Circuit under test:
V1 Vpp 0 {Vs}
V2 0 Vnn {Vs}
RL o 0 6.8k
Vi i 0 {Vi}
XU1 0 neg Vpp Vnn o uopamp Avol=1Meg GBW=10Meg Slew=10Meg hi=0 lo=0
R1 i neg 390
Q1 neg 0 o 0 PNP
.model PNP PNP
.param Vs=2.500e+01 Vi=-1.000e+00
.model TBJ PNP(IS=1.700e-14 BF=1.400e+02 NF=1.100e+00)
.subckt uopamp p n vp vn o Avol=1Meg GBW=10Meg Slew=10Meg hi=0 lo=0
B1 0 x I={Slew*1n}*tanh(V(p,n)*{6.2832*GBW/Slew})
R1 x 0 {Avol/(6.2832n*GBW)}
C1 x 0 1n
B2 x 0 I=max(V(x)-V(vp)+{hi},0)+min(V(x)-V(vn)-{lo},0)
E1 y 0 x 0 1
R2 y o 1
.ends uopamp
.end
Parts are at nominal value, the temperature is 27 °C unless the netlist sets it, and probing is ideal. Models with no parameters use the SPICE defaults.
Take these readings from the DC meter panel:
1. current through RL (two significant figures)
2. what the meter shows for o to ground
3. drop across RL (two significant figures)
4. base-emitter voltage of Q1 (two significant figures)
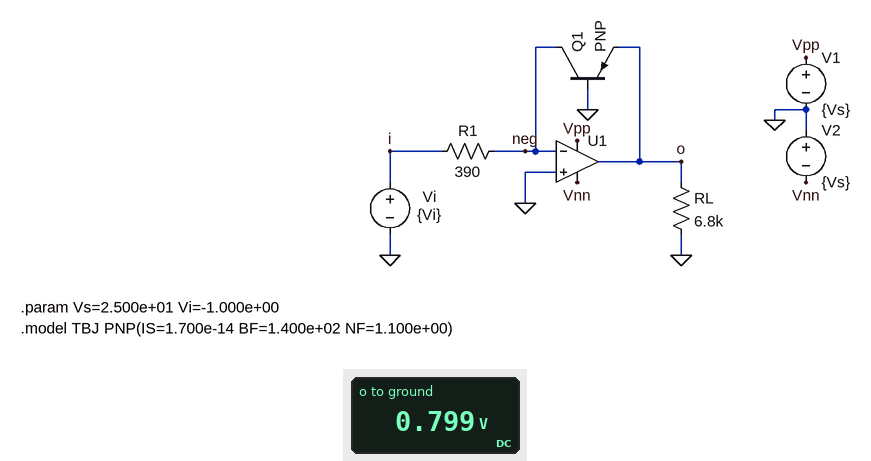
120 µA
0.799 V
800 mV
-800 mV
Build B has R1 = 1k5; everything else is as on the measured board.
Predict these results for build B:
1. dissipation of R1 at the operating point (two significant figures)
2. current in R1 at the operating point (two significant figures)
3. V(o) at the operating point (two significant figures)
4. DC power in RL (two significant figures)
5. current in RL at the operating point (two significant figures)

670 µW
670 µA
760 mV
86 µW
110 µA
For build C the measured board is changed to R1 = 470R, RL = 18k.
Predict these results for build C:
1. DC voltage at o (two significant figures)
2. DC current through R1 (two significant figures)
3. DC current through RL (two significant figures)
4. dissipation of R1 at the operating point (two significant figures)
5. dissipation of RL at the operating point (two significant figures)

790 mV
2.1 mA
44 µA
2.1 mW
35 µW
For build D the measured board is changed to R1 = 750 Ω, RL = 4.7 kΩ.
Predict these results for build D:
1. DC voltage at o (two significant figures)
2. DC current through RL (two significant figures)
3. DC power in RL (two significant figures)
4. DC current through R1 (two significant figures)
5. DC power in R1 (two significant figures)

780 mV
170 µA
130 µW
1.3 mA
1.3 mW
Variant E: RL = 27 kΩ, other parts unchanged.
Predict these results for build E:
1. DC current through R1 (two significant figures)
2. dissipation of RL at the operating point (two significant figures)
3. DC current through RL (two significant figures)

2.6 mA
24 µW
30 µA
